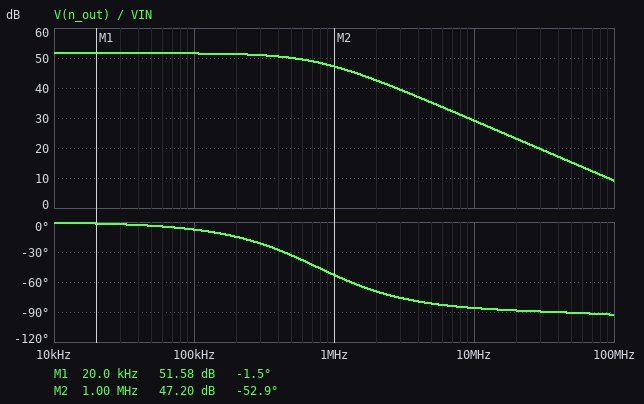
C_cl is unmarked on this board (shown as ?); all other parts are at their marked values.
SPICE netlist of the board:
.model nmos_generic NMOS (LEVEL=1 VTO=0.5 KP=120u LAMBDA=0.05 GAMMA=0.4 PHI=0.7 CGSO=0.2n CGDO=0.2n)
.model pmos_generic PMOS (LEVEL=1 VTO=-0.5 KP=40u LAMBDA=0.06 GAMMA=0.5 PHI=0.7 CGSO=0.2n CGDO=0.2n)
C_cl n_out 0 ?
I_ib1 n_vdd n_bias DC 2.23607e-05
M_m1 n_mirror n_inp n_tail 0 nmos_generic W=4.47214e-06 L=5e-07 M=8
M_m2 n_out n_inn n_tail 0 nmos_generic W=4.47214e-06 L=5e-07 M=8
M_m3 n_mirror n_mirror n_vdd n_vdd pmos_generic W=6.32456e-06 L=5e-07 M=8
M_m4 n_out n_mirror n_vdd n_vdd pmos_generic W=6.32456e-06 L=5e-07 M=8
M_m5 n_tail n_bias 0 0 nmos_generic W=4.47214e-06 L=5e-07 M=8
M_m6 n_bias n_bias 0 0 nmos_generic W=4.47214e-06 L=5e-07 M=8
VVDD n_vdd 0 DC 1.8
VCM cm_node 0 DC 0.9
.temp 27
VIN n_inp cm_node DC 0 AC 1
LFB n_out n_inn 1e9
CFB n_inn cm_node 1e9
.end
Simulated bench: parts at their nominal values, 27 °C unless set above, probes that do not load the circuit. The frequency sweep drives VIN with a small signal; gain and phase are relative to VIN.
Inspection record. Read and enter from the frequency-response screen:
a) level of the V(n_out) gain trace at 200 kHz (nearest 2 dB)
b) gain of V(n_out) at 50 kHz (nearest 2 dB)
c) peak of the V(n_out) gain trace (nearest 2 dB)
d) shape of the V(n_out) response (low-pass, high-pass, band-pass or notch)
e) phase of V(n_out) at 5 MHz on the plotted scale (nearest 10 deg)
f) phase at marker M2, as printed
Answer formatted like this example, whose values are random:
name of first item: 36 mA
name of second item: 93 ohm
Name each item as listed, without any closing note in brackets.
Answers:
level of the V(n_out) gain trace at 200 kHz: 52 dB
gain of V(n_out) at 50 kHz: 52 dB
peak of the V(n_out) gain trace: 52 dB
shape of the V(n_out) response: low-pass
phase of V(n_out) at 5 MHz on the plotted scale: -80 deg
phase at marker M2, as printed: -52.9 deg
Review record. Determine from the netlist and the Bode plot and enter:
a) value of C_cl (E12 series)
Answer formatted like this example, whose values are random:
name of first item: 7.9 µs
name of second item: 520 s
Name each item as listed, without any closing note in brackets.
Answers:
value of C_cl: 220 fF
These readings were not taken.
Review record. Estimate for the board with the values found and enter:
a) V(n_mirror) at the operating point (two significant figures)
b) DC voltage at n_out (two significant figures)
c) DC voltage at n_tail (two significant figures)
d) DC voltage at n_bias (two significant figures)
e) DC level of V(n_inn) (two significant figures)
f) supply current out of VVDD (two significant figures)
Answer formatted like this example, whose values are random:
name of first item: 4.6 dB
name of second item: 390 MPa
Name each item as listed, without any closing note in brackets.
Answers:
V(n_mirror) at the operating point: 1.2 V
DC voltage at n_out: 900 mV
DC voltage at n_tail: 290 mV
DC voltage at n_bias: 570 mV
DC level of V(n_inn): 900 mV
supply current out of VVDD: 44 µA
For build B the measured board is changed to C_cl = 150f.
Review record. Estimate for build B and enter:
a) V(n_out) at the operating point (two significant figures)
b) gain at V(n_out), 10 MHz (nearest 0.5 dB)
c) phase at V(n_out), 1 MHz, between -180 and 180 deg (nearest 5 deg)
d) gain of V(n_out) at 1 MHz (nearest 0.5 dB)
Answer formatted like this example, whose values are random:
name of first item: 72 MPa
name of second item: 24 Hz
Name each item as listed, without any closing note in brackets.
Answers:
V(n_out) at the operating point: 900 mV
gain at V(n_out), 10 MHz: 32.0 dB
phase at V(n_out), 1 MHz, between -180 and 180 deg: -45 deg
gain of V(n_out) at 1 MHz: 49.0 dB
